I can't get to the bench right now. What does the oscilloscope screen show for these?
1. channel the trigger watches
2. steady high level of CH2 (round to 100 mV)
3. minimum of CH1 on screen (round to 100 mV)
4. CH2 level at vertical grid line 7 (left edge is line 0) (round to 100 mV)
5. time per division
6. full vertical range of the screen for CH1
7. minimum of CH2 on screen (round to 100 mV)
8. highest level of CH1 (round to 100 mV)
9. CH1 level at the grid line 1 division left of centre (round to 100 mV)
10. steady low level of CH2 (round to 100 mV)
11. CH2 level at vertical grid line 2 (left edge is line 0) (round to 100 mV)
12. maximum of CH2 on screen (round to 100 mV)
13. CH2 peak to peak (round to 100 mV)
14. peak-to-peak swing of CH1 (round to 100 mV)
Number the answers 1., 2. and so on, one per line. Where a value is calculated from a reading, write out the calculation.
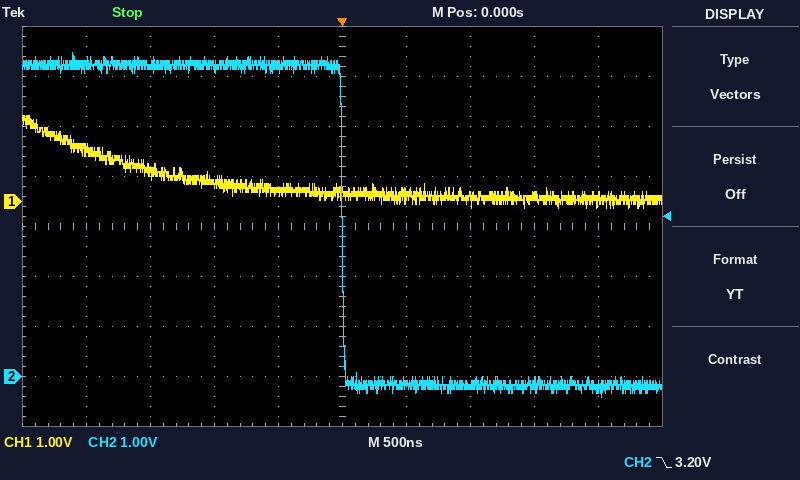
1. CH2
2. 6.2 V
3. -100 mV
4. -200 mV
5. 500 ns
6. 8 V
7. -400 mV
8. 1.7 V
9. 200 mV
10. -200 mV
11. 6.2 V
12. 6.5 V
13. 6.5 V − (-400 mV) = 6.9 V
14. 1.7 V − (-100 mV) = 1.8 V
